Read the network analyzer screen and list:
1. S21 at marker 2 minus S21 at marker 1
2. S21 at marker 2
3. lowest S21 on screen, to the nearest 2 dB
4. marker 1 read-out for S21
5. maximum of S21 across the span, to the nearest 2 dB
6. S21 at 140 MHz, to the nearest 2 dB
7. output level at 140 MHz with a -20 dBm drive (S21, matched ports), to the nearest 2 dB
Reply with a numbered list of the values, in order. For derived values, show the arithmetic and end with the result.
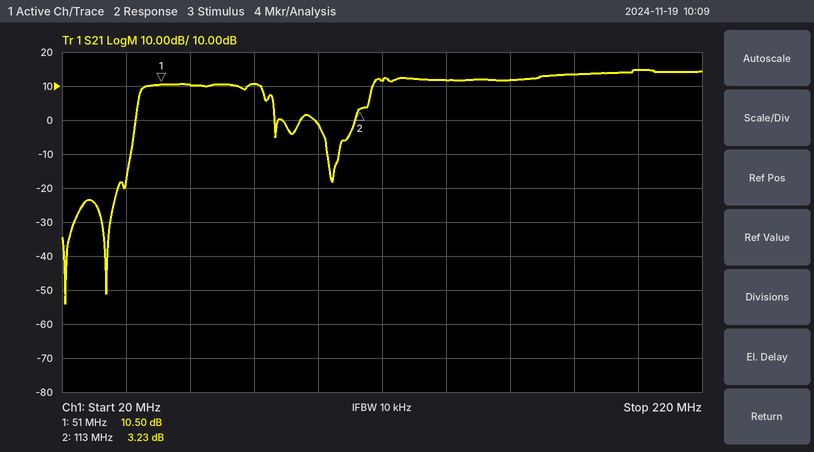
1. 3.23 − (10.5) = -7.27 dB
2. 3.23 dB
3. -54 dB
4. 10.50 dB
5. 14 dB
6. 12 dB
7. -20 dBm + (12 dB) = -8 dBm
